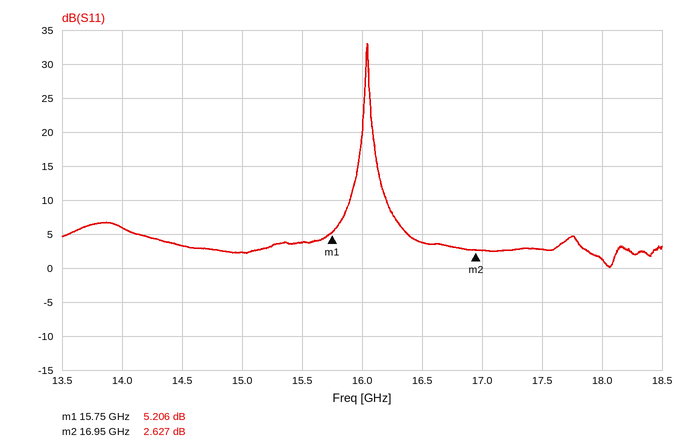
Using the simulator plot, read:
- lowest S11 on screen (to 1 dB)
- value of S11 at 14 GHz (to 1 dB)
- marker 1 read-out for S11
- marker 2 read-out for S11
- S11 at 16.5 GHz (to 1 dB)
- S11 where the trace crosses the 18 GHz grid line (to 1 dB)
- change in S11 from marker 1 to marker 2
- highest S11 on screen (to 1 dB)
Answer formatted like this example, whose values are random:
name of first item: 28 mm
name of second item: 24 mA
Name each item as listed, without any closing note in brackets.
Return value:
lowest S11 on screen: 0 dB
value of S11 at 14 GHz: 6 dB
marker 1 read-out for S11: 5.206 dB
marker 2 read-out for S11: 2.627 dB
S11 at 16.5 GHz: 4 dB
S11 where the trace crosses the 18 GHz grid line: 1 dB
change in S11 from marker 1 to marker 2: -2.579 dB
highest S11 on screen: 33 dB
